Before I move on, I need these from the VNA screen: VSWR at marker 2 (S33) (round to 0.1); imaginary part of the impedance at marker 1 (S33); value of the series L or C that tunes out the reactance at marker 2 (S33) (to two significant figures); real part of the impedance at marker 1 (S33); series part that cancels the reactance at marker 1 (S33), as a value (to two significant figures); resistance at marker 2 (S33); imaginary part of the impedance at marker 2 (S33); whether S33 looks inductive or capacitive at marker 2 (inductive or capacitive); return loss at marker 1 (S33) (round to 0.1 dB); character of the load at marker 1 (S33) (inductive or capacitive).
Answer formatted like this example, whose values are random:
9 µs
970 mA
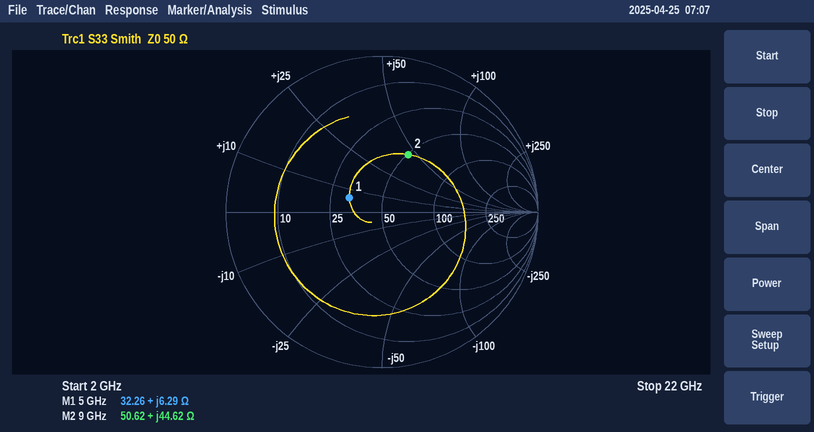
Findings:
2.4
+6.29 Ω
400 fF
32.26 Ω
5.1 pF
50.62 Ω
+44.62 Ω
inductive
12.8 dB
inductive
